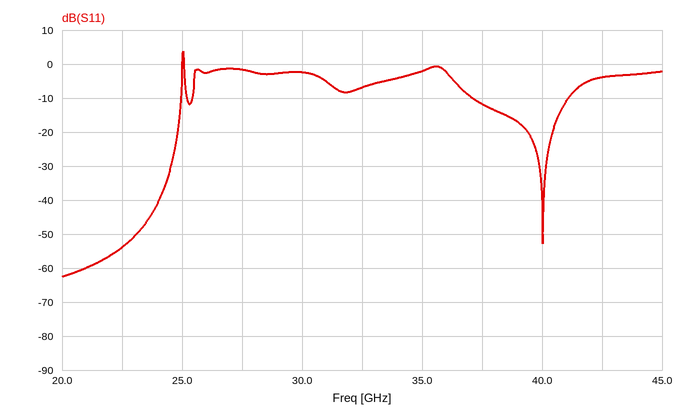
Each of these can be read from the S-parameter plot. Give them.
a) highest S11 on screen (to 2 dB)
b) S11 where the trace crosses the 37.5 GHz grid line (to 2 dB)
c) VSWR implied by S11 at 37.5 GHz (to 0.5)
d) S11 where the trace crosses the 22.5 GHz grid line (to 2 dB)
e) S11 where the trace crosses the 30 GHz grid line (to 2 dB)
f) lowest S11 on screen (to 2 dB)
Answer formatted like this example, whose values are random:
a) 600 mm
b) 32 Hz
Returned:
a) 4 dB
b) -12 dB
c) 1.5
d) -54 dB
e) -2 dB
f) -62 dB
